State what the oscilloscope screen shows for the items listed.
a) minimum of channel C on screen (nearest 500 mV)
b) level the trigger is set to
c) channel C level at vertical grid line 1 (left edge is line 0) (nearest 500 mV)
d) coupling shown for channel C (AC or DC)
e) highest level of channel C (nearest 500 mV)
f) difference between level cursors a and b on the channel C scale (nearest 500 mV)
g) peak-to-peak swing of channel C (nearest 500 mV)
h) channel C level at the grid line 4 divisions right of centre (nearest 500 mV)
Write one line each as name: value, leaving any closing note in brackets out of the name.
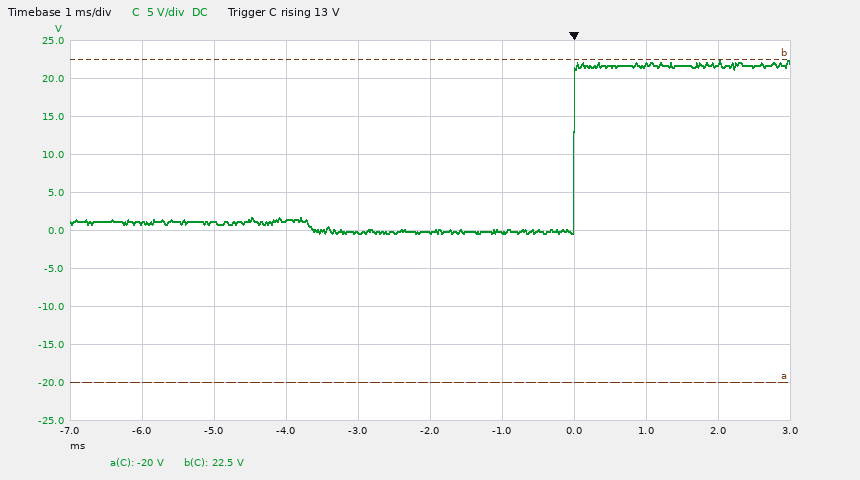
minimum of channel C on screen: -500 mV
level the trigger is set to: 13 V
channel C level at vertical grid line 1 (left edge is line 0): 1.0 V
coupling shown for channel C: DC
highest level of channel C: 22.5 V
difference between level cursors a and b on the channel C scale: 42.5 V
peak-to-peak swing of channel C: 23.0 V
channel C level at the grid line 4 divisions right of centre: 22.0 V
